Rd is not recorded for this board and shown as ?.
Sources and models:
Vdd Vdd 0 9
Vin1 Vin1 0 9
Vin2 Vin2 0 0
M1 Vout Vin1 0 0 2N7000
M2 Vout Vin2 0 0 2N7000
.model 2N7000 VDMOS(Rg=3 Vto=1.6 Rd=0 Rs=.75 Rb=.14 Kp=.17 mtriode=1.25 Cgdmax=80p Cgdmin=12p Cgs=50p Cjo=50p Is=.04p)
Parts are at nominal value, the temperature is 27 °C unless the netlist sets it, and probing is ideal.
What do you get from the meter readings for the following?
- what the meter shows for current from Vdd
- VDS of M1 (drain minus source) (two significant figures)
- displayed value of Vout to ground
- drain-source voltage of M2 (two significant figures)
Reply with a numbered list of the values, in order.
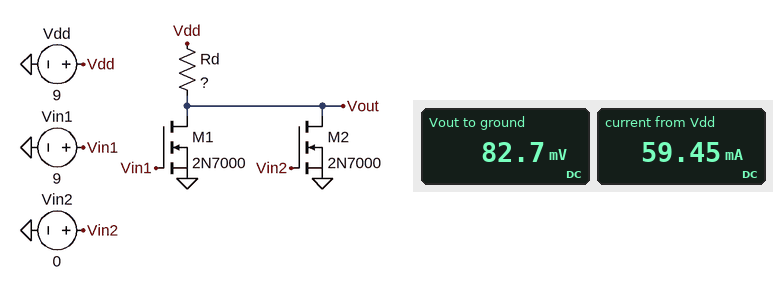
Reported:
1. 59.45 mA
2. 83 mV
3. 82.7 mV
4. 83 mV
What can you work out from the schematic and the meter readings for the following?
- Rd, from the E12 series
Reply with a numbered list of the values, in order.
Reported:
1. 150 Ω
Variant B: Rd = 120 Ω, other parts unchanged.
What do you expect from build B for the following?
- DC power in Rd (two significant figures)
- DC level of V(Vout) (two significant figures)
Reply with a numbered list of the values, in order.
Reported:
1. 660 mW
2. 100 mV
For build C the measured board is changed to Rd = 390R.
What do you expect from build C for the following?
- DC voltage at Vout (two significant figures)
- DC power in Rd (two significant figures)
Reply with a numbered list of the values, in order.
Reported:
1. 32 mV
2. 210 mW
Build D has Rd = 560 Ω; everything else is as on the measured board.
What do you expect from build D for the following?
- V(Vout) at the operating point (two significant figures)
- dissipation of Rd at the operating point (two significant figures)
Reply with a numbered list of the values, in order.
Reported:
1. 22 mV
2. 140 mW
